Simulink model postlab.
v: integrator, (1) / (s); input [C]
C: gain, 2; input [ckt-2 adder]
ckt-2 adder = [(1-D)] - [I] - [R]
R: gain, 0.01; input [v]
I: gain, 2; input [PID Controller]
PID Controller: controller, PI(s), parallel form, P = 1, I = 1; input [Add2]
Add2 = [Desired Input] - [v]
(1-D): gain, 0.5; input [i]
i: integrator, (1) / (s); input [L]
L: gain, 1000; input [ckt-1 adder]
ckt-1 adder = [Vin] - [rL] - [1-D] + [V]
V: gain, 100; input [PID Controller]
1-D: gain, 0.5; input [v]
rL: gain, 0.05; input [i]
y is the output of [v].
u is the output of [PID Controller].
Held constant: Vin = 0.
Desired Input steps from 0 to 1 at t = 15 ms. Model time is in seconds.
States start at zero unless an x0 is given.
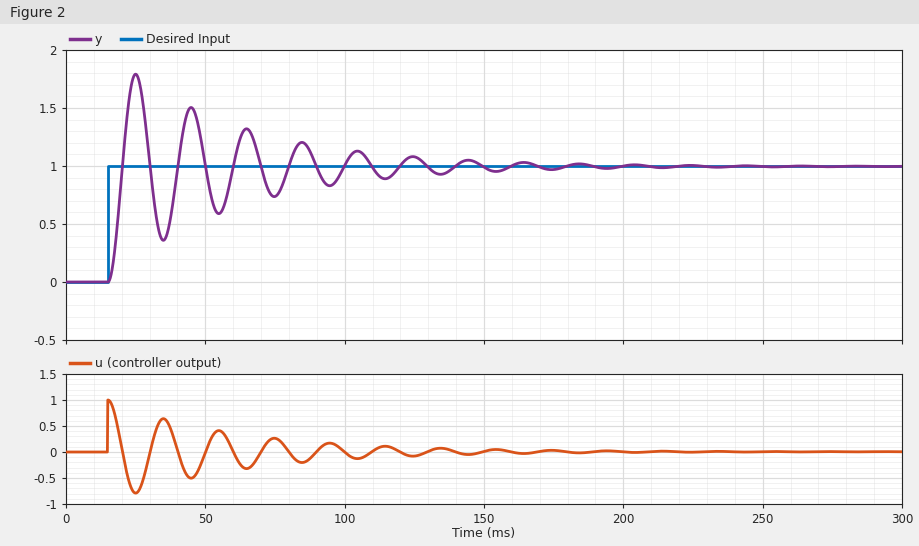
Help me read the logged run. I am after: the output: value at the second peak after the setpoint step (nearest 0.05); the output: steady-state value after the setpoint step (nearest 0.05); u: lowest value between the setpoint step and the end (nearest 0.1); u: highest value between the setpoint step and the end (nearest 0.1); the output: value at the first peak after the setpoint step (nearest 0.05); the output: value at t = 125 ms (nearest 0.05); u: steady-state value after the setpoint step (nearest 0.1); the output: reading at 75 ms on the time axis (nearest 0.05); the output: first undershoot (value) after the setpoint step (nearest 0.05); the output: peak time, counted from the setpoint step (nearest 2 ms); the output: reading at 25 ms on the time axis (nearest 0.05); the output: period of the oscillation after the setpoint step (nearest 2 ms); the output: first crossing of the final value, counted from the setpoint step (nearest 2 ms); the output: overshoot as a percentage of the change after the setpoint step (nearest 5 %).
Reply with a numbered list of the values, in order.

1. 1.50
2. 1.00
3. -0.8
4. 1.0
5. 1.80
6. 1.10
7. 0.0
8. 0.75
9. 0.35
10. 10 ms
11. 1.80
12. 20 ms
13. 6 ms
14. 80 %
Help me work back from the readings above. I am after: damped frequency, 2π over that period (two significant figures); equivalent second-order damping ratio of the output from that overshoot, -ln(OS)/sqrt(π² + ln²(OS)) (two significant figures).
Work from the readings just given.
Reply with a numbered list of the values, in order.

1. 0.31 rad/ms
2. 0.071
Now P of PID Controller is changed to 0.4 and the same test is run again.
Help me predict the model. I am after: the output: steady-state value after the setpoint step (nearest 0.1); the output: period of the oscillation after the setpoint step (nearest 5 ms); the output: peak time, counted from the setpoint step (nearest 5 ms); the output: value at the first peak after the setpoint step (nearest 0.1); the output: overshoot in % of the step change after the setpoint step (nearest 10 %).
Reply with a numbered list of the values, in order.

1. 1.0
2. 30 ms
3. 15 ms
4. 1.7
5. 70 %
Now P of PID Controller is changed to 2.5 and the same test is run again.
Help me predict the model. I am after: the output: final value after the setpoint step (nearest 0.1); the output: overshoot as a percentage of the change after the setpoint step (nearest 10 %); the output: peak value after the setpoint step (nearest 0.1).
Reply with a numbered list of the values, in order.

1. 1.0
2. 90 %
3. 1.9
